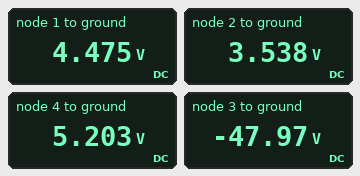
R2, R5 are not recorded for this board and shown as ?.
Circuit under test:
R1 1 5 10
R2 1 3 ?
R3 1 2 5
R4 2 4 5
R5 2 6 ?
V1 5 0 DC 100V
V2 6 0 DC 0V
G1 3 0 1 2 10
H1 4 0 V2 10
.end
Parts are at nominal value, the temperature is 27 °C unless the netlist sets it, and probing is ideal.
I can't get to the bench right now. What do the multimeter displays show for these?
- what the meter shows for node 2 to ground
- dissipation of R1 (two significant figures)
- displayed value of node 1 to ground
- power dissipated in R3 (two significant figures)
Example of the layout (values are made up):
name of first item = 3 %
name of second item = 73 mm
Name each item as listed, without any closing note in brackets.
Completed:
what the meter shows for node 2 to ground = 3.538 V
dissipation of R1 = 910 W
displayed value of node 1 to ground = 4.475 V
power dissipated in R3 = 180 mW
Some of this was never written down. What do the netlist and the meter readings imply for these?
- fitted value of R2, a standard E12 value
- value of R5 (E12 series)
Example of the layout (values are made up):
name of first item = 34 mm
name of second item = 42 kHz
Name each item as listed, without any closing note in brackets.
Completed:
fitted value of R2, a standard E12 value = 5.6 Ω
value of R5 = 6.8 Ω
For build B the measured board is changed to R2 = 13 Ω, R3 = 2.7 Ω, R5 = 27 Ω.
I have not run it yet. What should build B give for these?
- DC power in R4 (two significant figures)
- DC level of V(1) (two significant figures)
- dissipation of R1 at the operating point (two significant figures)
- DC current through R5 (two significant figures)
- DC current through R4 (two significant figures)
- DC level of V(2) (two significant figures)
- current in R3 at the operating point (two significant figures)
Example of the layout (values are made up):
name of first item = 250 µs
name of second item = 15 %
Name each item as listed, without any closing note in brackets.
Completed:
DC power in R4 = 360 mW
DC level of V(1) = 3.1 V
dissipation of R1 at the operating point = 940 W
DC current through R5 = 79 mA
DC current through R4 = 270 mA
DC level of V(2) = 2.1 V
current in R3 at the operating point = 350 mA
